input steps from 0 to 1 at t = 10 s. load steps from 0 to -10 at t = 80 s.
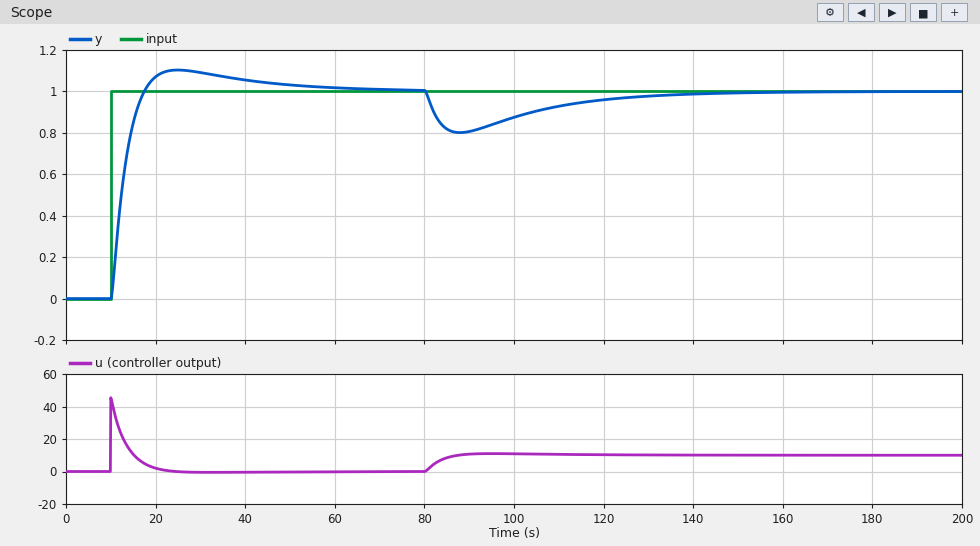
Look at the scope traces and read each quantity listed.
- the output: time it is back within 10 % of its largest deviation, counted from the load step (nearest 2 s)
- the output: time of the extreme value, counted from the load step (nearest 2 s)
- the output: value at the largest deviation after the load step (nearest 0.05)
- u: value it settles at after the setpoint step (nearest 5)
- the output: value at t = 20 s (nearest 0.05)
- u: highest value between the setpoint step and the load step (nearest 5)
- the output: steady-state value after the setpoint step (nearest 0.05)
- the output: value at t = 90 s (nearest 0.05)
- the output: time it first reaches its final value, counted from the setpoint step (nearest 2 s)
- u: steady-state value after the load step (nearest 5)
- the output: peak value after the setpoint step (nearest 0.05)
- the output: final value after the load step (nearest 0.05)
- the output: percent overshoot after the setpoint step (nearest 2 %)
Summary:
52 s
8 s
0.80
0
1.05
45
1.00
0.80
8 s
10
1.10
1.00
10 %
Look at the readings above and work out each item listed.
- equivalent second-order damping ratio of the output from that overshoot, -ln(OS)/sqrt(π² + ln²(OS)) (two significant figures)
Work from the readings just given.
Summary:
0.59
